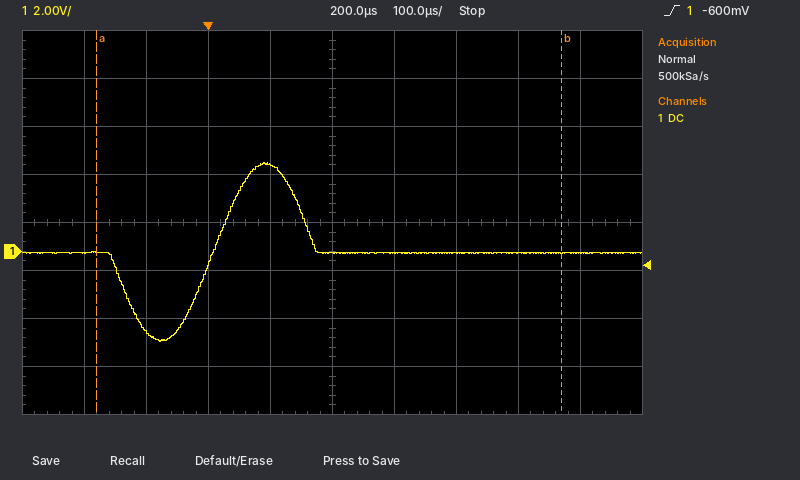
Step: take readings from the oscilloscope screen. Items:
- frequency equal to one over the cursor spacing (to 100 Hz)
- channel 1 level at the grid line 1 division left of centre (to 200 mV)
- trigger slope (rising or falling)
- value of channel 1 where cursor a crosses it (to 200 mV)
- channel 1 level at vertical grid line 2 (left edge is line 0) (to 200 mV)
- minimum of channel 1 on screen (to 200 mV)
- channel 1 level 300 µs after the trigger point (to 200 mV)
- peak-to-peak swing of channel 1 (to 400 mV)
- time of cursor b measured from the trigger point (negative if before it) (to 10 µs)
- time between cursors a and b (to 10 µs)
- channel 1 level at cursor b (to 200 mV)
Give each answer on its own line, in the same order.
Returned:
1.3 kHz
3.6 V
rising
0.0 V
-3.4 V
-3.8 V
0.0 V
7.6 V
+570 µs
750 µs
0.0 V
